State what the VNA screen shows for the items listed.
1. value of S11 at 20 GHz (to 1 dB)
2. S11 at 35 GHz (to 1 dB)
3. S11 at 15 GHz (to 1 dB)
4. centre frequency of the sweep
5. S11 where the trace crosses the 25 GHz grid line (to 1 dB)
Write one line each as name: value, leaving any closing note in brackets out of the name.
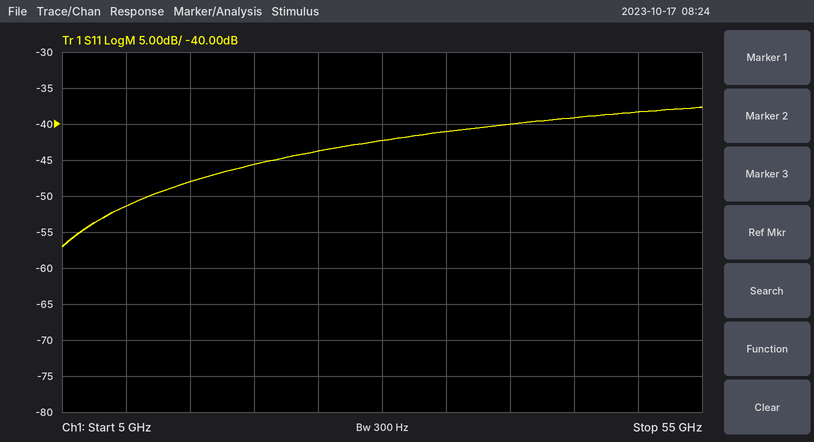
value of S11 at 20 GHz: -46 dB
S11 at 35 GHz: -41 dB
S11 at 15 GHz: -48 dB
centre frequency of the sweep: 30 GHz
S11 where the trace crosses the 25 GHz grid line: -44 dB
